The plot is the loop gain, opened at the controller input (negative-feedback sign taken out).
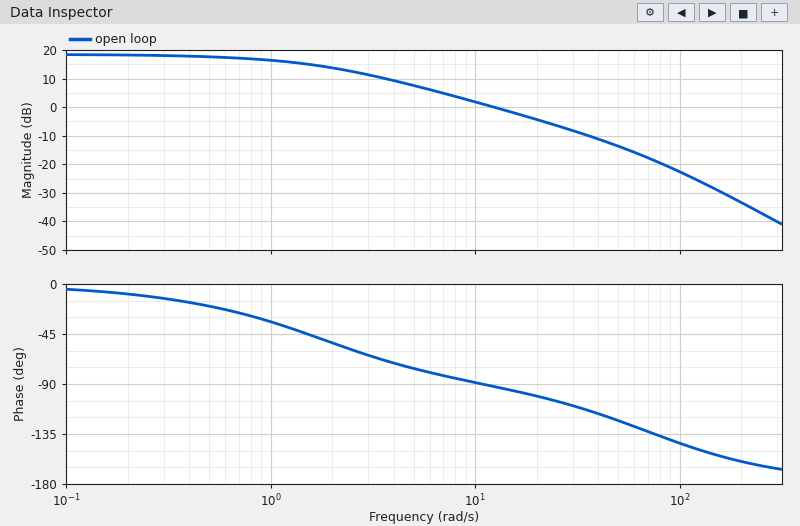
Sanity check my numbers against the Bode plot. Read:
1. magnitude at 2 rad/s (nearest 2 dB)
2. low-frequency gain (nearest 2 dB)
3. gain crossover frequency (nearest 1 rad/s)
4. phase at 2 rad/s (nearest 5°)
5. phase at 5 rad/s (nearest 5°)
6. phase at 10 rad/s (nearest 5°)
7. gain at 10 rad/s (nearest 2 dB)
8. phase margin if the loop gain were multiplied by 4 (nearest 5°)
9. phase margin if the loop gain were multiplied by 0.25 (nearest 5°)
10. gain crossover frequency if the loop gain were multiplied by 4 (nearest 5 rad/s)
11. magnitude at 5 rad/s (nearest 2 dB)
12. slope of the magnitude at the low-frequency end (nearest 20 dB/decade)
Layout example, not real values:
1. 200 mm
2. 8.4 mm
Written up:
1. 14 dB
2. 18 dB
3. 12 rad/s
4. -55°
5. -75°
6. -90°
7. 2 dB
8. 60°
9. 120°
10. 45 rad/s
11. 8 dB
12. 0 dB/decade
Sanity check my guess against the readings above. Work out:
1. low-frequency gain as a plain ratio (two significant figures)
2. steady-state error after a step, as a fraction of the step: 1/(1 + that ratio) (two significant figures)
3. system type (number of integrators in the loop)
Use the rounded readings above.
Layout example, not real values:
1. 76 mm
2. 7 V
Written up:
1. 7.9
2. 0.11
3. 0
